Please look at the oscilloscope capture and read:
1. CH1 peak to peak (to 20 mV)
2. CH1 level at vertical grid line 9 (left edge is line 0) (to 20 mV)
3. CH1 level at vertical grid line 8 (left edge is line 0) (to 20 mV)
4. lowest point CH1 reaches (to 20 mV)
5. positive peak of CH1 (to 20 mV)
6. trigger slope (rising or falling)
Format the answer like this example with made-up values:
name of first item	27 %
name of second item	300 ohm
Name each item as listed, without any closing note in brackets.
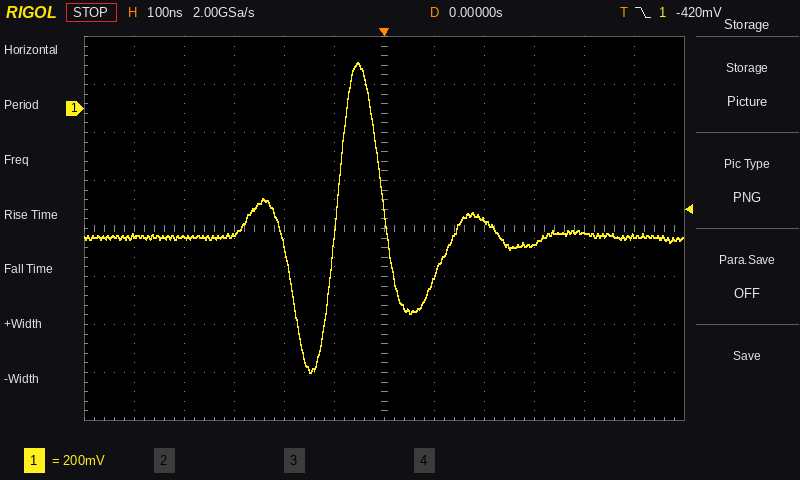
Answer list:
CH1 peak to peak	1.30 V
CH1 level at vertical grid line 9 (left edge is line 0)	-560 mV
CH1 level at vertical grid line 8 (left edge is line 0)	-460 mV
lowest point CH1 reaches	-1.10 V
positive peak of CH1	200 mV
trigger slope	falling
